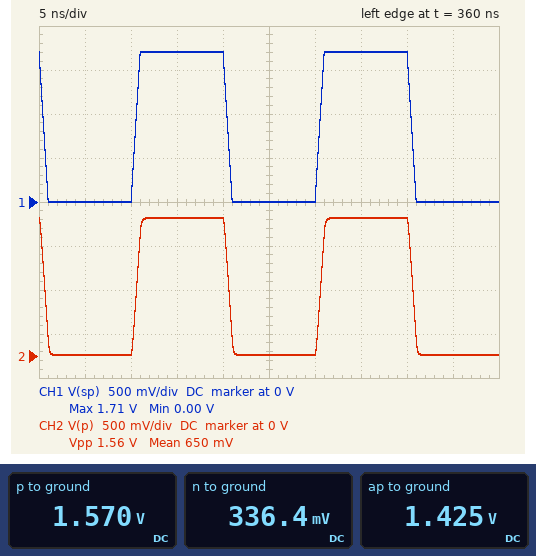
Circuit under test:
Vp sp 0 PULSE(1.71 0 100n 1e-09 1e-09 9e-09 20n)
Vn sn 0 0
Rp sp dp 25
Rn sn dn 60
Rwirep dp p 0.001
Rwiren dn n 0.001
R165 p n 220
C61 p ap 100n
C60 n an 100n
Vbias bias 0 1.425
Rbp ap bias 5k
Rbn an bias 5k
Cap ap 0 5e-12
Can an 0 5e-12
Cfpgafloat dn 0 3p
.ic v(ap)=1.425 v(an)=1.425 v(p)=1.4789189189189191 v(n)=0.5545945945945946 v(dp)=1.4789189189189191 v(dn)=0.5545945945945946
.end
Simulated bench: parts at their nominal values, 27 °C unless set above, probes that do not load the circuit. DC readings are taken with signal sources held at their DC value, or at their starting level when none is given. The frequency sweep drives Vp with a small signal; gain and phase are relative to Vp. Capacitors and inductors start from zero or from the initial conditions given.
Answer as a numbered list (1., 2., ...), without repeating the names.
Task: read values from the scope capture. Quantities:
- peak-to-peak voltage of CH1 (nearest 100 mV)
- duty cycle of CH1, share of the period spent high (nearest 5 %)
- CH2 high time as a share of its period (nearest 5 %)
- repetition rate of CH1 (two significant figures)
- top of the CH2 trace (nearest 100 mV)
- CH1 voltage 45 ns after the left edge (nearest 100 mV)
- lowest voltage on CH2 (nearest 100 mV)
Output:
1. 1.7 V
2. 50 %
3. 50 %
4. 50 MHz
5. 1.6 V
6. 0 V
7. 0 V
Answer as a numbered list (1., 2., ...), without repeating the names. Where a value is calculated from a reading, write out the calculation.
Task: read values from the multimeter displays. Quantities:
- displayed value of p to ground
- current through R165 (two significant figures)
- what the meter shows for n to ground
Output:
1. 1.570 V
2. (1.57 V - 336.4 mV) / 220 Ω = 5.6 mA
3. 336.4 mV
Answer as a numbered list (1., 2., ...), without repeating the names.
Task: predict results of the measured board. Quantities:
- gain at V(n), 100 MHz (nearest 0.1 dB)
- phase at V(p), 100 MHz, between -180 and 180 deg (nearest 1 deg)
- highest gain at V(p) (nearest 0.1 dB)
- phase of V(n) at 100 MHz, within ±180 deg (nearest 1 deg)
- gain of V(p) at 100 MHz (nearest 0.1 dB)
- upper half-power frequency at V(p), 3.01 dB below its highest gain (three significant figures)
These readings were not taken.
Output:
1. -14.5 dB
2. -4 deg
3. -0.8 dB
4. -18 deg
5. -0.8 dB
6. 1.36 GHz
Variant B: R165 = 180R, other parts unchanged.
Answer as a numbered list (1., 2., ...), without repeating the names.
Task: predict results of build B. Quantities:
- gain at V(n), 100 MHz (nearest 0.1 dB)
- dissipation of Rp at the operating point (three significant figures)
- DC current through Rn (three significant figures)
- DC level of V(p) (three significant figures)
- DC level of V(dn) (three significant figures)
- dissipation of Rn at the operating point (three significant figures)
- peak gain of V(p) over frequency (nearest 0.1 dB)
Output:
1. -13.3 dB
2. 1.04 mW
3. 6.45 mA
4. 1.55 V
5. 387 mV
6. 2.50 mW
7. -0.9 dB
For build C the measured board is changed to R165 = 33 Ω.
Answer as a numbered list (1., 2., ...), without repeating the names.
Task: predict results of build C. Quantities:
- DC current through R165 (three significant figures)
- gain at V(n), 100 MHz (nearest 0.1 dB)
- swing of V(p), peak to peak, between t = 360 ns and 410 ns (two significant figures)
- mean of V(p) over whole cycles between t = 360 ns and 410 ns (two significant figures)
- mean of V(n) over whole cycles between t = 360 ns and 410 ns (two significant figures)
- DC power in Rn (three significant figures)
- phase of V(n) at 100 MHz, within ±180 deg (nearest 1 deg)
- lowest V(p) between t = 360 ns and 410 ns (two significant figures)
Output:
1. 14.5 mA
2. -6.1 dB
3. 1.3 V
4. 680 mV
5. 440 mV
6. 12.6 mW
7. -12 deg
8. 7.2 mV
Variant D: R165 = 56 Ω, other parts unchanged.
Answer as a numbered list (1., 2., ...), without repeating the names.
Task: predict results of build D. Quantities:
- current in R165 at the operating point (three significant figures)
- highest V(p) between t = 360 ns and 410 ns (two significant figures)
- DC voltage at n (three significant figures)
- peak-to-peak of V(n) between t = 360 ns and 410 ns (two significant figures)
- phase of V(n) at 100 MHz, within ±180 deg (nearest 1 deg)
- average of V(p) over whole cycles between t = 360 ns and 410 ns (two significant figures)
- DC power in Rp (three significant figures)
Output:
1. 12.1 mA
2. 1.4 V
3. 728 mV
4. 720 mV
5. -13 deg
6. 710 mV
7. 3.68 mW
